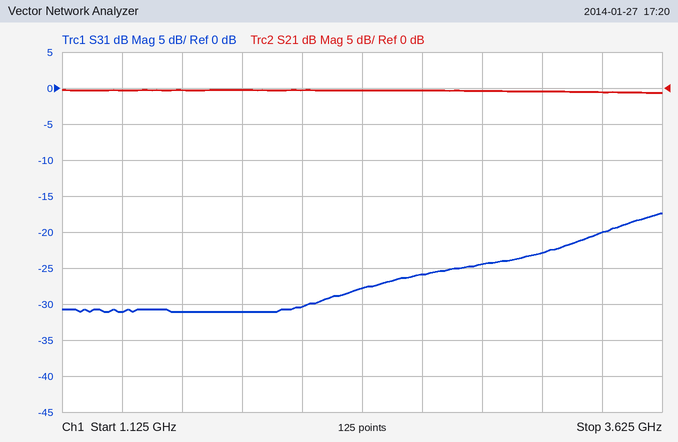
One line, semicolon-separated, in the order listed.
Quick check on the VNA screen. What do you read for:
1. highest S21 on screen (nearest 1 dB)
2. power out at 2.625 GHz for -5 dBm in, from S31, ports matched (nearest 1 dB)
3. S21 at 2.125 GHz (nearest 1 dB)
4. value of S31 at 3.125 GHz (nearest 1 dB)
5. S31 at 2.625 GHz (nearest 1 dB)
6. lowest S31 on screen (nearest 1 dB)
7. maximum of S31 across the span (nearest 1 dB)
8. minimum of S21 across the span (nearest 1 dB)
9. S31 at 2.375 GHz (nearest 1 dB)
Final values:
0 dB; -31 dBm; 0 dB; -23 dB; -26 dB; -31 dB; -17 dB; -1 dB; -28 dB
